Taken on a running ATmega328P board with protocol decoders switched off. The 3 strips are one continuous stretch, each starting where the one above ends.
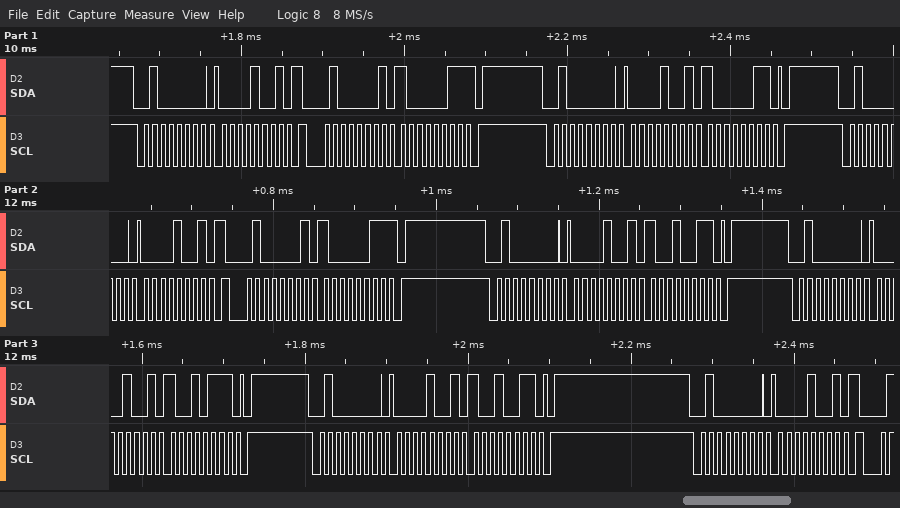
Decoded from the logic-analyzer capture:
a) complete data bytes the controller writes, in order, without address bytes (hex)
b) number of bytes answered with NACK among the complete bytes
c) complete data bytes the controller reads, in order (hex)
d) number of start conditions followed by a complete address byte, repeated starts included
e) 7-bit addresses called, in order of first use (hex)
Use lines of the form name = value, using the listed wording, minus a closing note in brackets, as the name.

complete data bytes the controller writes, in order, without address bytes = 09 09 83 09 09 93 09 97 09 93 09
number of bytes answered with NACK among the complete bytes = 2
complete data bytes the controller reads, in order = 83 83
number of start conditions followed by a complete address byte, repeated starts included = 9
7-bit addresses called, in order of first use = 0x20
